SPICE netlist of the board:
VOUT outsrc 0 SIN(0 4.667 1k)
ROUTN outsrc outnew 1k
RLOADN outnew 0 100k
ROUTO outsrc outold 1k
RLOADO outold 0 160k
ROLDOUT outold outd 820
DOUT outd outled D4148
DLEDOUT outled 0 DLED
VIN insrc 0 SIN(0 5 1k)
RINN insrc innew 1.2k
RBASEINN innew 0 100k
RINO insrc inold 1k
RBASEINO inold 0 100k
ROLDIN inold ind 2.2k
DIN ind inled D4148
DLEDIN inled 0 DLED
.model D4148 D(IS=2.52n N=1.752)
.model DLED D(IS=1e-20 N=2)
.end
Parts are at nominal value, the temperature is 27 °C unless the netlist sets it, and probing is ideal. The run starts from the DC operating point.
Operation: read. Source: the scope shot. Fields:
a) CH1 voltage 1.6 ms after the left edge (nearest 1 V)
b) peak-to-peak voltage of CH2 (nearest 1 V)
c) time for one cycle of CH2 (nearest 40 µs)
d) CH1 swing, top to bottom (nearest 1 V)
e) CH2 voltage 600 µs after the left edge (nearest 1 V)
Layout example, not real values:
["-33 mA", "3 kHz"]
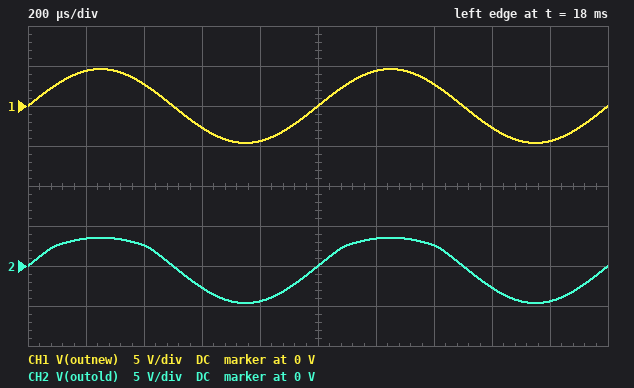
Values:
["-3 V", "8 V", "1.00 ms", "9 V", "-3 V"]
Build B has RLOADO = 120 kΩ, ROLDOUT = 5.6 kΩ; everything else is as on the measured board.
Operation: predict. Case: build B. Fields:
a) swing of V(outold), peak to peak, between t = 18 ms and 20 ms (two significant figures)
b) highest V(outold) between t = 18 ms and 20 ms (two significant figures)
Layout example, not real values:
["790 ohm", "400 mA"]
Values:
["8.9 V", "4.3 V"]
